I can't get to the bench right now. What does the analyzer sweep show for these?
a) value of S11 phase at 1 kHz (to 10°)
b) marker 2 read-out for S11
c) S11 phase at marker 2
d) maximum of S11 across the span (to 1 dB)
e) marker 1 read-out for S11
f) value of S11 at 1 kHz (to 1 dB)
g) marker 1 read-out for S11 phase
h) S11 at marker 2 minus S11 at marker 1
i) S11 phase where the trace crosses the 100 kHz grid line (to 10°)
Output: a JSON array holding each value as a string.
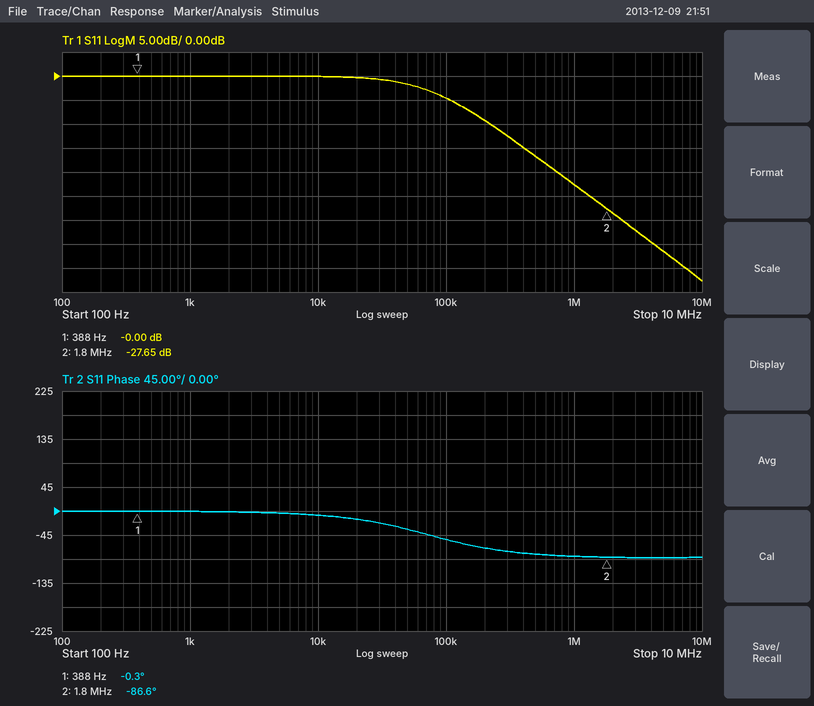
["0°", "-27.65 dB", "-86.6°", "0 dB", "-0.00 dB", "0 dB", "-0.3°", "-27.65 dB", "-50°"]
